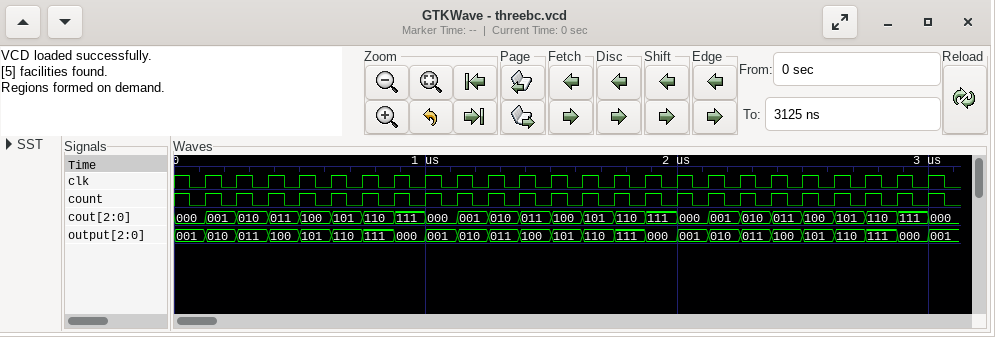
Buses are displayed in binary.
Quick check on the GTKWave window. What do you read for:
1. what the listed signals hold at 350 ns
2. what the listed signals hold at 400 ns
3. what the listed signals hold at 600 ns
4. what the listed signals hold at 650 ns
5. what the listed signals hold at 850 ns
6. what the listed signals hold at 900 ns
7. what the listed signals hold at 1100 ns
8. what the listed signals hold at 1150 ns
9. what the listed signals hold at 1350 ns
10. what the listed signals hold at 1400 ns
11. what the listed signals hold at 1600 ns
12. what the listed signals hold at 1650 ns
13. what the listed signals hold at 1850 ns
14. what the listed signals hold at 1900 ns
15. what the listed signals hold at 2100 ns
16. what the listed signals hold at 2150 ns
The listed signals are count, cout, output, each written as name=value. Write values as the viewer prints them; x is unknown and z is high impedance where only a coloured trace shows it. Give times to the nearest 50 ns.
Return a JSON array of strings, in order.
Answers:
["count=0, cout=010, output=011", "count=1, cout=011, output=100", "count=0, cout=100, output=101", "count=1, cout=101, output=110", "count=0, cout=110, output=111", "count=1, cout=111, output=000", "count=0, cout=000, output=001", "count=1, cout=001, output=010", "count=0, cout=010, output=011", "count=1, cout=011, output=100", "count=0, cout=100, output=101", "count=1, cout=101, output=110", "count=0, cout=110, output=111", "count=1, cout=111, output=000", "count=0, cout=000, output=001", "count=1, cout=001, output=010"]
